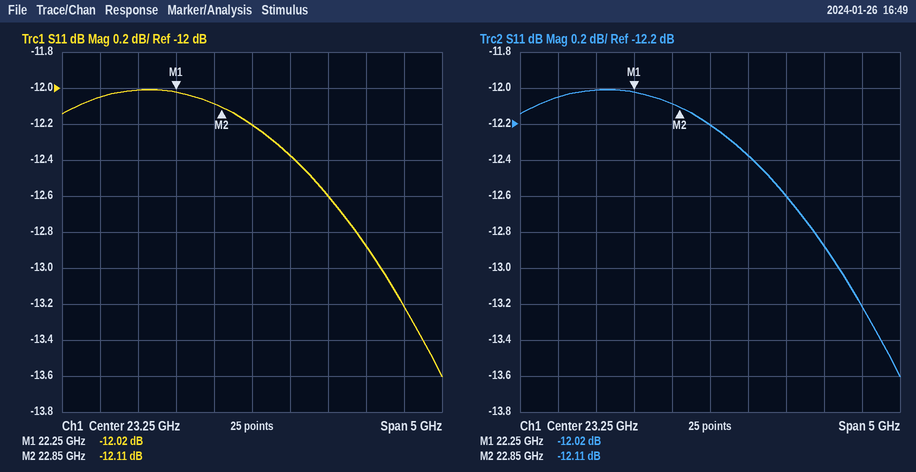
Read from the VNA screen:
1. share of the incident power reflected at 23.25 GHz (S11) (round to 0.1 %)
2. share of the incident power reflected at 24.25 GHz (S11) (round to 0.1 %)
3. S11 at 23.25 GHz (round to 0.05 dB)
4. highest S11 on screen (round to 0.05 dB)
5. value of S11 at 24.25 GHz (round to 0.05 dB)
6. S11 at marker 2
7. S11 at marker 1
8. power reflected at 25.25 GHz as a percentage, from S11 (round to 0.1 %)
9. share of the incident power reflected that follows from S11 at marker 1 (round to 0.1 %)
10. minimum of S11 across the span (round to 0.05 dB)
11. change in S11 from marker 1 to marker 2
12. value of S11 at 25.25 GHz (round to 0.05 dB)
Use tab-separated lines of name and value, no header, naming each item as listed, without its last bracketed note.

share of the incident power reflected at 23.25 GHz (S11)	6.0 %
share of the incident power reflected at 24.25 GHz (S11)	5.5 %
S11 at 23.25 GHz	-12.20 dB
highest S11 on screen	-12.00 dB
value of S11 at 24.25 GHz	-12.60 dB
S11 at marker 2	-12.11 dB
S11 at marker 1	-12.02 dB
power reflected at 25.25 GHz as a percentage, from S11	4.8 %
share of the incident power reflected that follows from S11 at marker 1	6.3 %
minimum of S11 across the span	-13.60 dB
change in S11 from marker 1 to marker 2	-0.09 dB
value of S11 at 25.25 GHz	-13.20 dB
